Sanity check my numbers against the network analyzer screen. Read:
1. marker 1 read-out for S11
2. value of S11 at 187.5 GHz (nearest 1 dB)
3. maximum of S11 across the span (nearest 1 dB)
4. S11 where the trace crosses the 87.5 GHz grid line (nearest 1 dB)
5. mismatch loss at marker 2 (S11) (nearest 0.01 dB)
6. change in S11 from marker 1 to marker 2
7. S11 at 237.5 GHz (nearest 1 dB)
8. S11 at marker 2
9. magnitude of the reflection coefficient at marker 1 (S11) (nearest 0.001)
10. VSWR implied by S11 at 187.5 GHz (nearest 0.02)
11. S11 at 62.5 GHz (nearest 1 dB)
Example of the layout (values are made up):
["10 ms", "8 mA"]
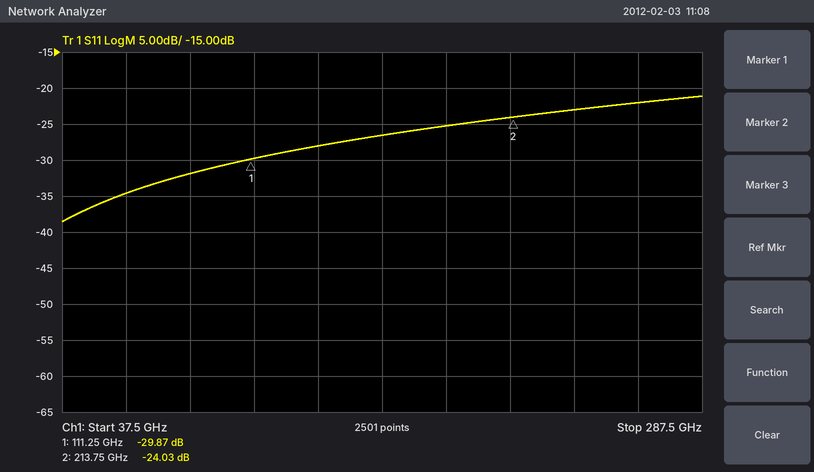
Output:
["-29.87 dB", "-25 dB", "-21 dB", "-32 dB", "0.02 dB", "5.84 dB", "-23 dB", "-24.03 dB", "0.032", "1.12", "-35 dB"]
